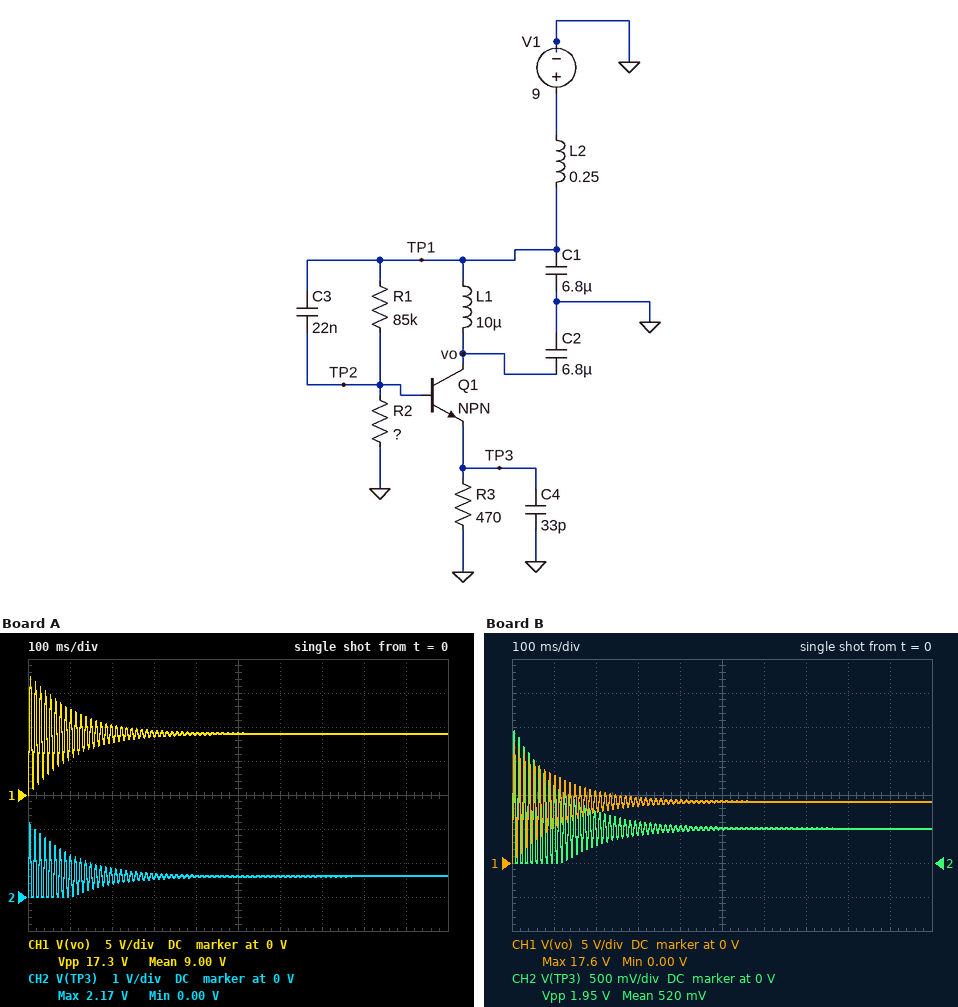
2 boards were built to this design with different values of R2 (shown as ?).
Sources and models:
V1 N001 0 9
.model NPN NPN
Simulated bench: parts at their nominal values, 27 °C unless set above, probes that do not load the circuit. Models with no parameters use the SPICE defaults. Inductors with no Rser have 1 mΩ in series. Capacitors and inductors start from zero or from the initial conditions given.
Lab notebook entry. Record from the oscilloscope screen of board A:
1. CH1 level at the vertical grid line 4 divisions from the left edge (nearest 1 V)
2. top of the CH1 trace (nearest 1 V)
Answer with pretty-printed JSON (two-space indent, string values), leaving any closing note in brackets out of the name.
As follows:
{
  "CH1 level at the vertical grid line 4 divisions from the left edge": "9 V",
  "top of the CH1 trace": "17 V"
}
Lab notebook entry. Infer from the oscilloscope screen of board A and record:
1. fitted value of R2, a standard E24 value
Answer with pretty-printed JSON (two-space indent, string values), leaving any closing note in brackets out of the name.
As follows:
{
  "fitted value of R2, a standard E24 value": "18 kΩ"
}
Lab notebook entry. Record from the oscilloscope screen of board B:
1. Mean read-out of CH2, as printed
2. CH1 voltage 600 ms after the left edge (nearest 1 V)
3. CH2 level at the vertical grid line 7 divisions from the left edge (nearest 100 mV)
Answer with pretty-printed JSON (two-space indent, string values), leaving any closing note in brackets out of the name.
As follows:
{
  "Mean read-out of CH2, as printed": "520 mV",
  "CH1 voltage 600 ms after the left edge": "9 V",
  "CH2 level at the vertical grid line 7 divisions from the left edge": "500 mV"
}
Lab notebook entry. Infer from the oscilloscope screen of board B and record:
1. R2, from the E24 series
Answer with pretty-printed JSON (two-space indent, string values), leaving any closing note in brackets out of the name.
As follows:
{
  "R2, from the E24 series": "16 kΩ"
}
